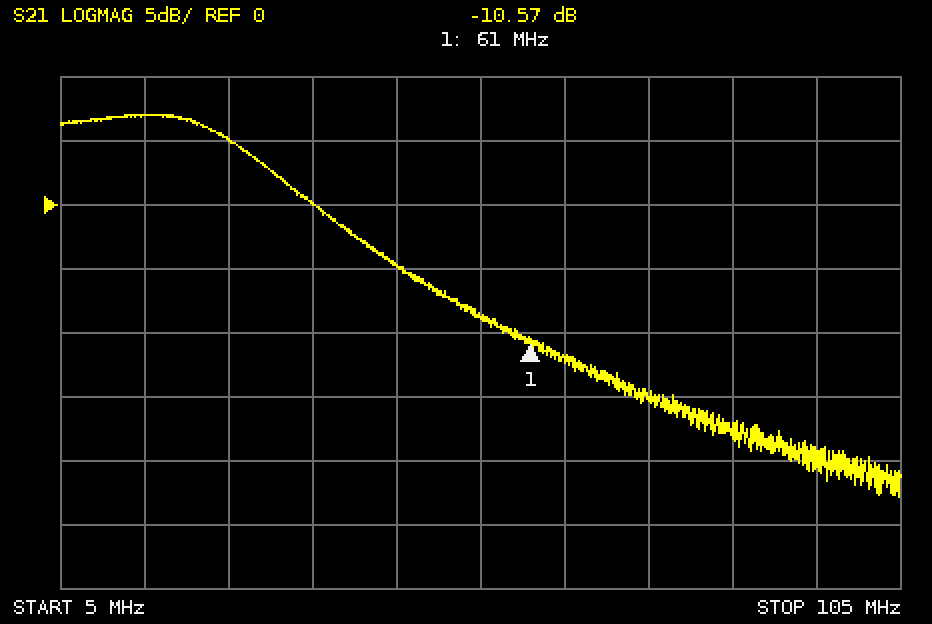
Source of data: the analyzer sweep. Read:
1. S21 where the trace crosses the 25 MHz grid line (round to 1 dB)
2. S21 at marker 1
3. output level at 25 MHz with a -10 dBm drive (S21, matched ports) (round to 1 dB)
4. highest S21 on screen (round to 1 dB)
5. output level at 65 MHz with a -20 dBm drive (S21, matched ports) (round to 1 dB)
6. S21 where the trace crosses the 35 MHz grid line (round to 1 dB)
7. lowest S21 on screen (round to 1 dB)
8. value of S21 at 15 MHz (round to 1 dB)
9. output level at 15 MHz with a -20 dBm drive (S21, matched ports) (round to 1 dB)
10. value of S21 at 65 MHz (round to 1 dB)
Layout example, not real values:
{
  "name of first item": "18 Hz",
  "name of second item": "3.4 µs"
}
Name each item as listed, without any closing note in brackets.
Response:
{
  "S21 where the trace crosses the 25 MHz grid line": "5 dB",
  "S21 at marker 1": "-10.57 dB",
  "output level at 25 MHz with a -10 dBm drive (S21, matched ports)": "-5 dBm",
  "highest S21 on screen": "7 dB",
  "output level at 65 MHz with a -20 dBm drive (S21, matched ports)": "-32 dBm",
  "S21 where the trace crosses the 35 MHz grid line": "0 dB",
  "lowest S21 on screen": "-23 dB",
  "value of S21 at 15 MHz": "7 dB",
  "output level at 15 MHz with a -20 dBm drive (S21, matched ports)": "-13 dBm",
  "value of S21 at 65 MHz": "-12 dB"
}
